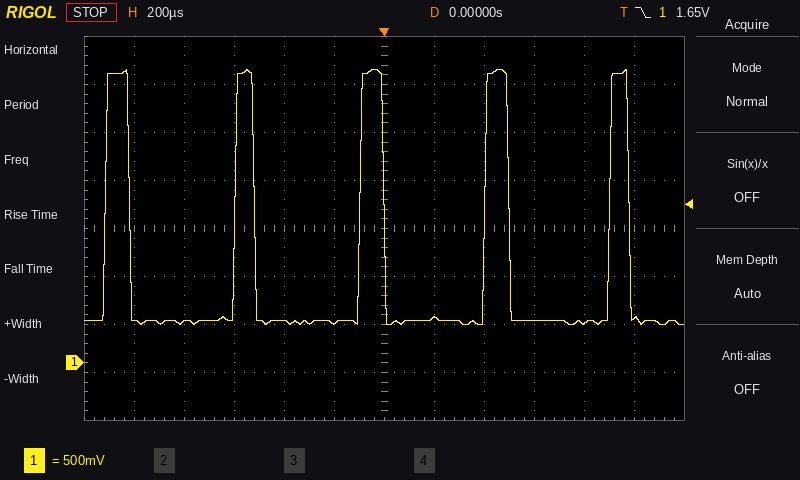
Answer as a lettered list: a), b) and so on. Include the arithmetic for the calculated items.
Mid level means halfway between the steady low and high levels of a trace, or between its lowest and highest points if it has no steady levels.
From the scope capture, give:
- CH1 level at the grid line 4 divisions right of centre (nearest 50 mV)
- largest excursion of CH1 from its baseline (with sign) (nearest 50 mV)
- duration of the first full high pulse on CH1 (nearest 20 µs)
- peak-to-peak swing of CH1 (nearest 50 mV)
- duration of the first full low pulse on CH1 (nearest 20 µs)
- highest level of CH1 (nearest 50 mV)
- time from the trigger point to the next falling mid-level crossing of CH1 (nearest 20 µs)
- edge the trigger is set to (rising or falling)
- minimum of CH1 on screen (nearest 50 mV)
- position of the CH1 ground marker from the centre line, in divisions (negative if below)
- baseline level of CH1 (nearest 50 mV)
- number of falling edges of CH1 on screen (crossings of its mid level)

a) 400 mV
b) 3.05 V − (450 mV) = +2.60 V
c) 100 µs
d) 3.05 V − (400 mV) = 2.65 V
e) 420 µs
f) 3.05 V
g) 500 µs
h) falling
i) 400 mV
j) -2.8 div
k) 450 mV
l) 5
